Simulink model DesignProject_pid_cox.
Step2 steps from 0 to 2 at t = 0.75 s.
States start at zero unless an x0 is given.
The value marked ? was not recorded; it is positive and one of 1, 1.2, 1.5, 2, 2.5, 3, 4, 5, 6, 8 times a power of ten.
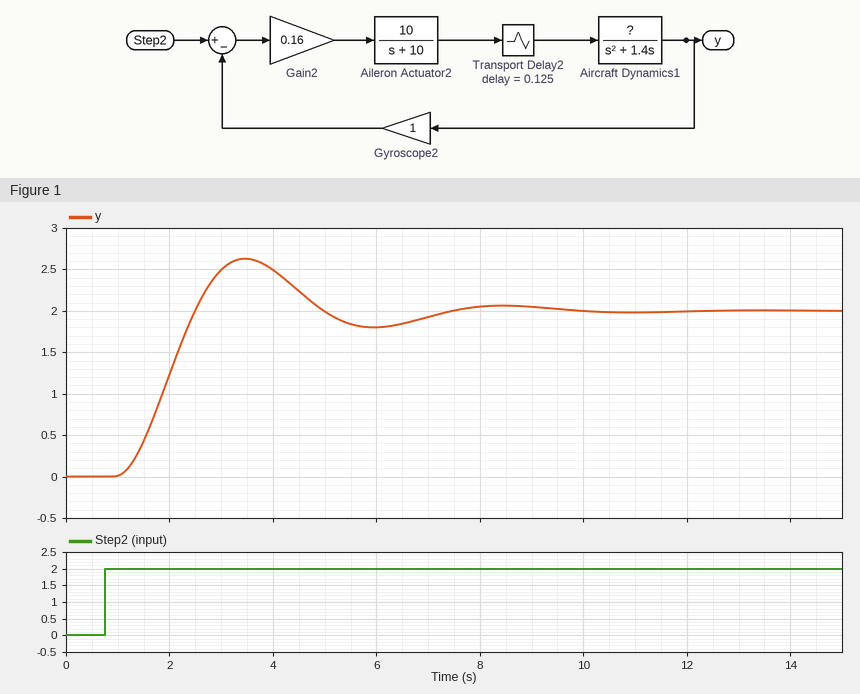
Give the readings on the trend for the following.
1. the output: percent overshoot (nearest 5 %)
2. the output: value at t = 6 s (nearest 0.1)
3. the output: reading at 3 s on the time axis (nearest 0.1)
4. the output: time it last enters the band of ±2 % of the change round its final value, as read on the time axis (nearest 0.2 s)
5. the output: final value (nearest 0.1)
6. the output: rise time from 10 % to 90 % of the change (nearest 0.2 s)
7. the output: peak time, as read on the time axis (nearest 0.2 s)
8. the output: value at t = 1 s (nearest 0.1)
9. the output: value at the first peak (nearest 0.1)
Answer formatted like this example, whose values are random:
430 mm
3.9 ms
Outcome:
30 %
1.8
2.5
9.2 s
2.0
1.0 s
3.4 s
0.0
2.6
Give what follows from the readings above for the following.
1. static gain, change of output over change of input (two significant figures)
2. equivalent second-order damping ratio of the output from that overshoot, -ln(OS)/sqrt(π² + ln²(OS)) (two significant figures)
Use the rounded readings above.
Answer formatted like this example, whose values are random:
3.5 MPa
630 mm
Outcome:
1.0
0.36
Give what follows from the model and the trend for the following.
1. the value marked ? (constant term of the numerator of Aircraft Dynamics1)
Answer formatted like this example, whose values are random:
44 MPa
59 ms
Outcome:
12
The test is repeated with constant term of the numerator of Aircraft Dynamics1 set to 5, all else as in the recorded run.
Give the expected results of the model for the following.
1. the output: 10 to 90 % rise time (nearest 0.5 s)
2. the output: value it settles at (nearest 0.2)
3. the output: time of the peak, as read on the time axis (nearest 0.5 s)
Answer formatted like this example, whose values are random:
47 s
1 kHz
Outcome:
2.5 s
2.0
6.0 s
